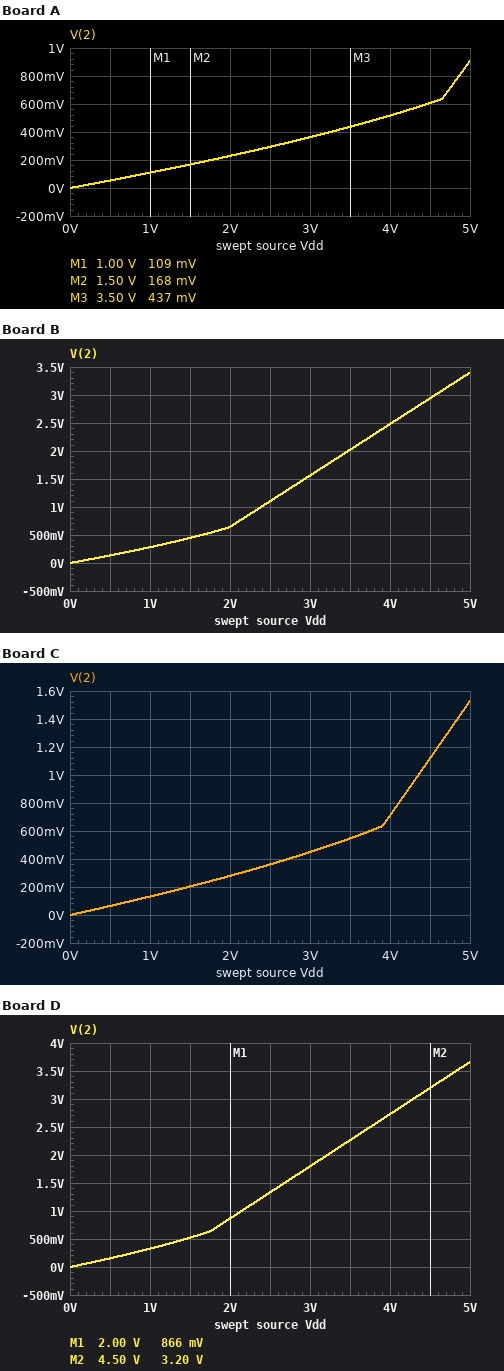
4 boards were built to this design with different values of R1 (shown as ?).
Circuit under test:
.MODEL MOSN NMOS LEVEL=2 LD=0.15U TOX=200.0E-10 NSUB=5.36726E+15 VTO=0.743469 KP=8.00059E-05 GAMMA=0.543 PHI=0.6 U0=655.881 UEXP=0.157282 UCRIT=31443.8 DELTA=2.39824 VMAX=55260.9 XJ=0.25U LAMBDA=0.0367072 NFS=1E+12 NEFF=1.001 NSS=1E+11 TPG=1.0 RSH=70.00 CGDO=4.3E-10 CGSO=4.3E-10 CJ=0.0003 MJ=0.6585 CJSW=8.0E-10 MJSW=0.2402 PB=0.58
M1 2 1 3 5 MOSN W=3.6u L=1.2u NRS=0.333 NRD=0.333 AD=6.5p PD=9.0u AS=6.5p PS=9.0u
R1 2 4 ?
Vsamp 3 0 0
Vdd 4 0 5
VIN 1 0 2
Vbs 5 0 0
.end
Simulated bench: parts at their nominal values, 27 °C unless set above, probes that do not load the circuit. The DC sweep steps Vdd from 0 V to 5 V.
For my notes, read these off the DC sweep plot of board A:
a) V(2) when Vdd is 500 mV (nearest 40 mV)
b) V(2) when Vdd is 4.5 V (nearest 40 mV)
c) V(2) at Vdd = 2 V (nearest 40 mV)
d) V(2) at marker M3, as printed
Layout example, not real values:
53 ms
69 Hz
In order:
40 mV
600 mV
240 mV
437 mV
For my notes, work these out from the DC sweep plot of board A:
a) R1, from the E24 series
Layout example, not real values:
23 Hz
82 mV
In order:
27 kΩ
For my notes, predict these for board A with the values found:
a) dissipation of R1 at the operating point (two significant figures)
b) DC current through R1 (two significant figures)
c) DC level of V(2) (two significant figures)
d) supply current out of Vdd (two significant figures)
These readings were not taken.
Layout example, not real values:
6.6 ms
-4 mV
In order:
620 µW
150 µA
910 mV
150 µA
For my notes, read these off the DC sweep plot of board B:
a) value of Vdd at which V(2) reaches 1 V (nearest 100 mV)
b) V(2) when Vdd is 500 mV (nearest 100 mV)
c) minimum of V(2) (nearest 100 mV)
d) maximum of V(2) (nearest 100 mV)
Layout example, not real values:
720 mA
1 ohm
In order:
2.4 V
100 mV
0 V
3.4 V
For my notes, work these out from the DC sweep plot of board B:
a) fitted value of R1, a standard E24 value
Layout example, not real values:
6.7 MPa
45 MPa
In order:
9.1 kΩ
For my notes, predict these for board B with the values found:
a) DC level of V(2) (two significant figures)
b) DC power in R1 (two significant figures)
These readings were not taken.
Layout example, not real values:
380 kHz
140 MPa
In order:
3.4 V
280 µW
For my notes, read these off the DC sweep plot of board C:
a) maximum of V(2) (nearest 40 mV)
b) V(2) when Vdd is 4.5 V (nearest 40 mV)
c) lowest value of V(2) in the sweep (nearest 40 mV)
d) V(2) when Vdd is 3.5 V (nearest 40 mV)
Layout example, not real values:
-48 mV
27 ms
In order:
1.52 V
1.12 V
0 V
560 mV
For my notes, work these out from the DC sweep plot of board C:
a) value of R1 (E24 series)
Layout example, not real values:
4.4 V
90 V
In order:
22 kΩ
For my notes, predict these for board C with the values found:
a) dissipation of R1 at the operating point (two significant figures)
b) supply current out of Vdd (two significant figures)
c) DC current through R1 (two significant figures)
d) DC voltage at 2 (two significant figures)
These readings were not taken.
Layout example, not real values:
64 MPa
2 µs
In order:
550 µW
160 µA
160 µA
1.5 V
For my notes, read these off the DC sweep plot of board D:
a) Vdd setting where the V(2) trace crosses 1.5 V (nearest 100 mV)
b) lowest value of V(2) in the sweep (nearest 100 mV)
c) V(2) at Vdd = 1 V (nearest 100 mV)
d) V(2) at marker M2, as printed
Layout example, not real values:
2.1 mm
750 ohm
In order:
2.7 V
0 V
300 mV
3.20 V
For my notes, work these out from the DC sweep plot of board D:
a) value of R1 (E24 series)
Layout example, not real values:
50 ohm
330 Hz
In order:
7.5 kΩ
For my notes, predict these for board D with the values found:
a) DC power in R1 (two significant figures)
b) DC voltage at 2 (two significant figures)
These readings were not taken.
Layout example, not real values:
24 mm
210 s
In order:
240 µW
3.7 V
